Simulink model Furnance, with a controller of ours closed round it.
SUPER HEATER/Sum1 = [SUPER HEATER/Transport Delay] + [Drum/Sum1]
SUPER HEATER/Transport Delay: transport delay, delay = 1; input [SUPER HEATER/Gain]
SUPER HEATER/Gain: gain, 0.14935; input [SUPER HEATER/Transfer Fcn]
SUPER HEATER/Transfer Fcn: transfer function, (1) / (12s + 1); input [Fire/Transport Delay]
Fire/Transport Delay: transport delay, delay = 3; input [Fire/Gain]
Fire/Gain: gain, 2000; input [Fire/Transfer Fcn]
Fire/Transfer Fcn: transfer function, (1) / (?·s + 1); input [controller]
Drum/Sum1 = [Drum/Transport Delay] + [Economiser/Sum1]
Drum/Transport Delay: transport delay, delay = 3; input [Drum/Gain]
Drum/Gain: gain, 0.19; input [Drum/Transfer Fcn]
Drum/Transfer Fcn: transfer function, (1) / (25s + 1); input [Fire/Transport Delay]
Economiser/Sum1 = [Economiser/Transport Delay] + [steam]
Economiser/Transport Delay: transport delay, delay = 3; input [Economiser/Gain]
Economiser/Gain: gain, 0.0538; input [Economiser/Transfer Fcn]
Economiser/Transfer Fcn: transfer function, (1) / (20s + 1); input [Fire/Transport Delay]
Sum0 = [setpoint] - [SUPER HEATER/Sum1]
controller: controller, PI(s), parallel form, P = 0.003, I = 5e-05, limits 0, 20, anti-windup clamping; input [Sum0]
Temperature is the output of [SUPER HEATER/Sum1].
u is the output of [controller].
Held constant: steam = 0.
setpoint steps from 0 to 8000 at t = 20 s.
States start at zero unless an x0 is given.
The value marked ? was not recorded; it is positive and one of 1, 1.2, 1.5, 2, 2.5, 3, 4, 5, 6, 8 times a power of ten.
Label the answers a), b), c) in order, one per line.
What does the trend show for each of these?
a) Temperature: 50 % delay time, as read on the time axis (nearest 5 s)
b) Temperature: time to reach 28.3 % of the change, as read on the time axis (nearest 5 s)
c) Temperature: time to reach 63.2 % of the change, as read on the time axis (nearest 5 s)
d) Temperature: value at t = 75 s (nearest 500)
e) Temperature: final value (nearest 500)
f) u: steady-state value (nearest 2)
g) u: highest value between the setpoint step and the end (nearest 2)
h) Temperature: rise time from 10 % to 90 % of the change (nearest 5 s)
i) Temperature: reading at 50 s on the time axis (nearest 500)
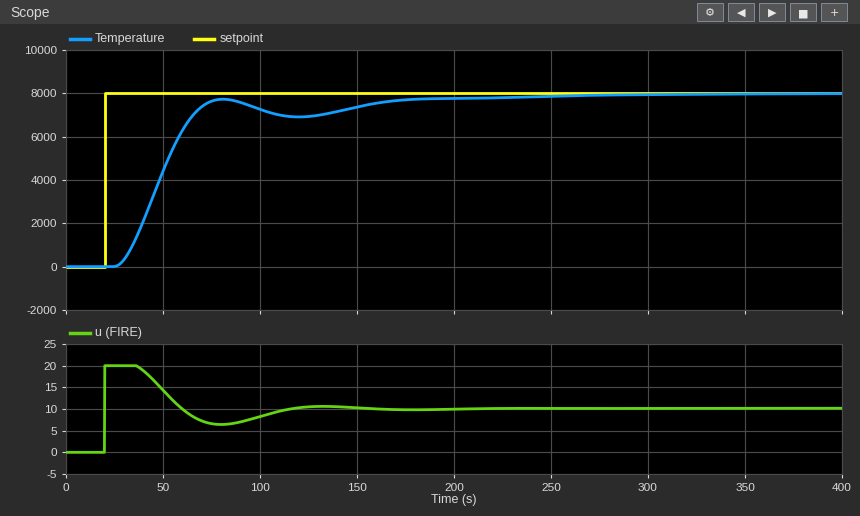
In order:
a) 50 s
b) 40 s
c) 55 s
d) 7500
e) 8000
f) 10
g) 20
h) 35 s
i) 4500
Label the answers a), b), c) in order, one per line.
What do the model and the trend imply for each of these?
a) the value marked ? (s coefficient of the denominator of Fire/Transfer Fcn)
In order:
a) 30
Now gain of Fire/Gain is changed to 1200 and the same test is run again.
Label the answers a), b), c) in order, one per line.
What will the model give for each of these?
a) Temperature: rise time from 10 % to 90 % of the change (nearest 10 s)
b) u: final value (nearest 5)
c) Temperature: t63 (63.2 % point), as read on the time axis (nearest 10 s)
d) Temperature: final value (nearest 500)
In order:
a) 130 s
b) 15
c) 70 s
d) 8000
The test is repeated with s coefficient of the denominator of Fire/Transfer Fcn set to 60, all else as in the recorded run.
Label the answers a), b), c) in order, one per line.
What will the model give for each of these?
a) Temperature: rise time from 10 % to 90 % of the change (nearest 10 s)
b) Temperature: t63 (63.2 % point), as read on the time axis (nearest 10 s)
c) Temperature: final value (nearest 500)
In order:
a) 50 s
b) 70 s
c) 8000
